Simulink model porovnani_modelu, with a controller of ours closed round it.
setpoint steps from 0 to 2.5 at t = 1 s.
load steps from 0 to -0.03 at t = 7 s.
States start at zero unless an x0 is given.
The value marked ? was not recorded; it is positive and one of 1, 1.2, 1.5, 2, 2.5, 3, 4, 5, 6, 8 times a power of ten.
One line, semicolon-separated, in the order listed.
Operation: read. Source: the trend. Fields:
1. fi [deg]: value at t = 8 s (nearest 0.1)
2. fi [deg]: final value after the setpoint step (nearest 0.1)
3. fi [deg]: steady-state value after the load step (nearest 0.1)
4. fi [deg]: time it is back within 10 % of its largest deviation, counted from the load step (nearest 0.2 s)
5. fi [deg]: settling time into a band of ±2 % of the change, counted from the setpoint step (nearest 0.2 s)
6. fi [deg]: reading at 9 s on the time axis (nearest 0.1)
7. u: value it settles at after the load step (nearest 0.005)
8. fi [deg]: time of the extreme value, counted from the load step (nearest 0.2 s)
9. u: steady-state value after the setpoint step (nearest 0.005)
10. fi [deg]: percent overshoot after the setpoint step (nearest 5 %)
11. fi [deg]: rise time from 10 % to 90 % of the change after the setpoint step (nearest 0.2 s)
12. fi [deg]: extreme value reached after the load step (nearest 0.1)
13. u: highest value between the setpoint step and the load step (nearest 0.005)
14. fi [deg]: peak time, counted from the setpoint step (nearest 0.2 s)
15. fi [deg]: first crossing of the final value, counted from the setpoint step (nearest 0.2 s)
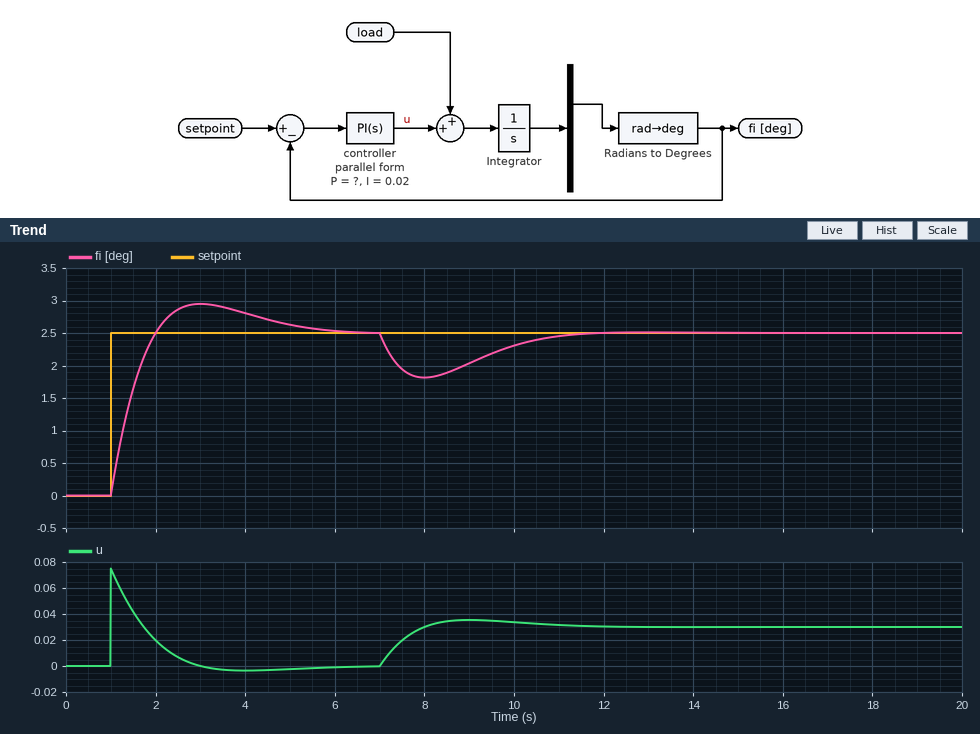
1.8; 2.5; 2.5; 3.8 s; 4.8 s; 2.0; 0.030; 1.0 s; 0.000; 20 %; 0.8 s; 1.8; 0.075; 2.0 s; 1.0 s
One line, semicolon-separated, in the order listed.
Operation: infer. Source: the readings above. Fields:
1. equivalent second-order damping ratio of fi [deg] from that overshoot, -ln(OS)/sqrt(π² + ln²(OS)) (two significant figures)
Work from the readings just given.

0.46
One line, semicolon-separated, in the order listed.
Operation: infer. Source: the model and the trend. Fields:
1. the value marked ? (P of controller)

0.03
